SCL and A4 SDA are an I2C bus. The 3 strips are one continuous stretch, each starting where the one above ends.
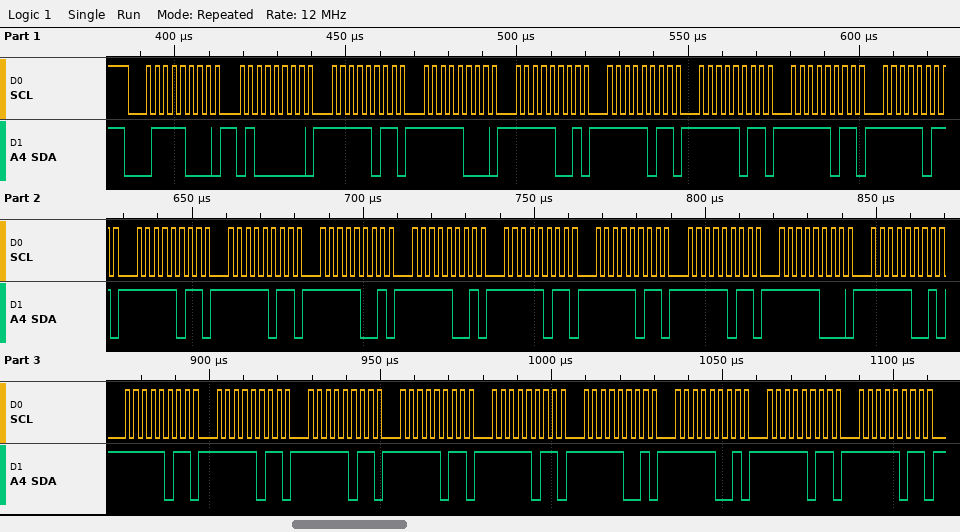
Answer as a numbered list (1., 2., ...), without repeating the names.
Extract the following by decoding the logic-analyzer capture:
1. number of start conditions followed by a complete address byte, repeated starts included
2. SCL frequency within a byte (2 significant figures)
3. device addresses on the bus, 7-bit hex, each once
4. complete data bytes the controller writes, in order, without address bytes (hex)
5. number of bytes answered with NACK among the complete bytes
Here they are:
1. 1
2. 400 kHz
3. 0x3C
4. 40 FB F8 F9 FB FB FB FB FB FB F9 F9 FB FB FB F8 F9 FB FB FB FB FB F9 F9 FB FB
5. 0
